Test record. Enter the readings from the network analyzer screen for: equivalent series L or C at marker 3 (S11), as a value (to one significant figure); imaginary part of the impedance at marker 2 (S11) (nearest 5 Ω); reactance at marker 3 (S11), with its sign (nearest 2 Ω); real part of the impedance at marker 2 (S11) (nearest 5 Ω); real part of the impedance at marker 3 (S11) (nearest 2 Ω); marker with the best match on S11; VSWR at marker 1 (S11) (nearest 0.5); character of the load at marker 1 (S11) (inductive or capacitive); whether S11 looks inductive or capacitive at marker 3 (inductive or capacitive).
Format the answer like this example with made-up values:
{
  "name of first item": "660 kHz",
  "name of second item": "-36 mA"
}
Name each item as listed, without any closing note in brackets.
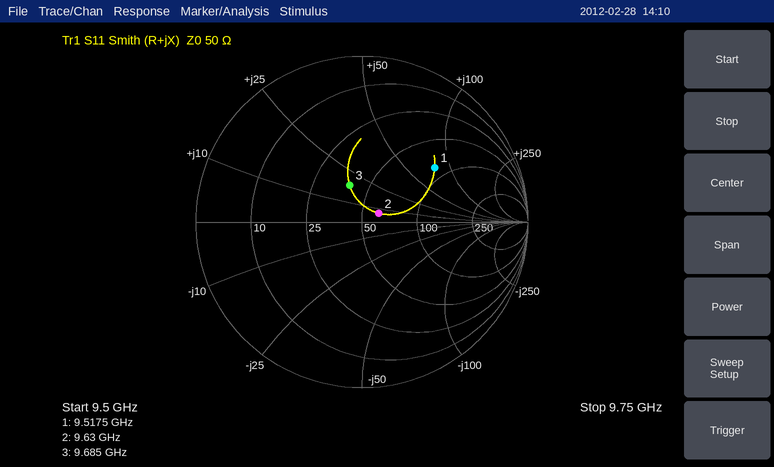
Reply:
{
  "equivalent series L or C at marker 3 (S11), as a value": "300 pH",
  "imaginary part of the impedance at marker 2 (S11)": "+5 Ω",
  "reactance at marker 3 (S11), with its sign": "+18 Ω",
  "real part of the impedance at marker 2 (S11)": "60 Ω",
  "real part of the impedance at marker 3 (S11)": "40 Ω",
  "marker with the best match on S11": "marker 2",
  "VSWR at marker 1 (S11)": "3.5",
  "character of the load at marker 1 (S11)": "inductive",
  "whether S11 looks inductive or capacitive at marker 3": "inductive"
}
